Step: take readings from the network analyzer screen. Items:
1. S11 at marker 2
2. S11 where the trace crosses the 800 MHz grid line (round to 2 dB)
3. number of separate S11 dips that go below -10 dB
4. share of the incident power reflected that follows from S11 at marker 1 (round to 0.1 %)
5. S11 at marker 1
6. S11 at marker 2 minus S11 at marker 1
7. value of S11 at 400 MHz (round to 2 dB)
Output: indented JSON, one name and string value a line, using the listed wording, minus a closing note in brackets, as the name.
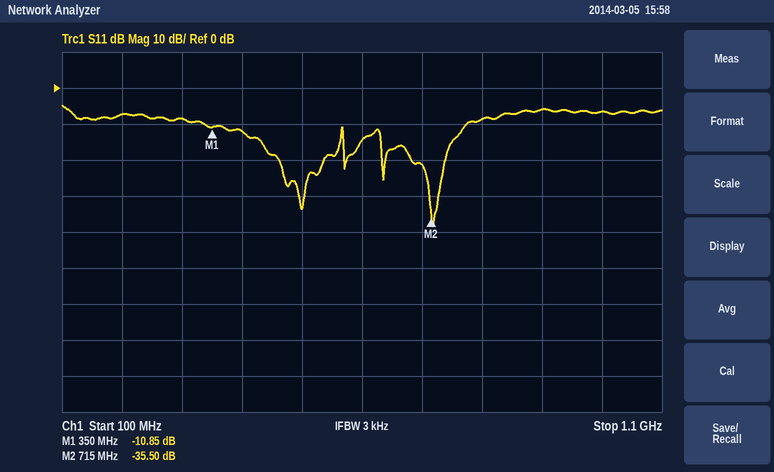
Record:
{
  "S11 at marker 2": "-35.50 dB",
  "S11 where the trace crosses the 800 MHz grid line": "-8 dB",
  "number of separate S11 dips that go below -10 dB": "4",
  "share of the incident power reflected that follows from S11 at marker 1": "8.2 %",
  "S11 at marker 1": "-10.85 dB",
  "S11 at marker 2 minus S11 at marker 1": "-24.65 dB",
  "value of S11 at 400 MHz": "-12 dB"
}
